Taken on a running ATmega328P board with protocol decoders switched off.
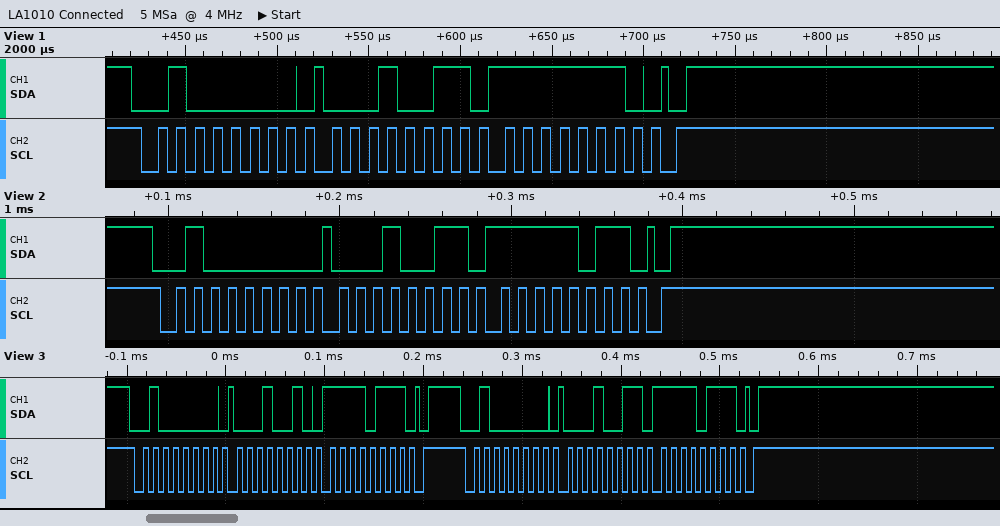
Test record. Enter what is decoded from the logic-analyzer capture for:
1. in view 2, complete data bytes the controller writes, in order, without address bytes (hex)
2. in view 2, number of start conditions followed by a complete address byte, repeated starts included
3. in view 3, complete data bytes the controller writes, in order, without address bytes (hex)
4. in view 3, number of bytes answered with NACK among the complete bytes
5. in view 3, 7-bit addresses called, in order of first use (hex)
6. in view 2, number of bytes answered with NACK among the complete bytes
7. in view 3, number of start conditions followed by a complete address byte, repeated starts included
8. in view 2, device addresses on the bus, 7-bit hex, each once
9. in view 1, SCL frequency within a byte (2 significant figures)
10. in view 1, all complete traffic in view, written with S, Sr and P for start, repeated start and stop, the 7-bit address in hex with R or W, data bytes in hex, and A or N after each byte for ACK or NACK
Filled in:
13 FB
1
12 F7 13 F7
0
0x20
0
2
0x20
100 kHz
S 20W A 13 A FE A P
